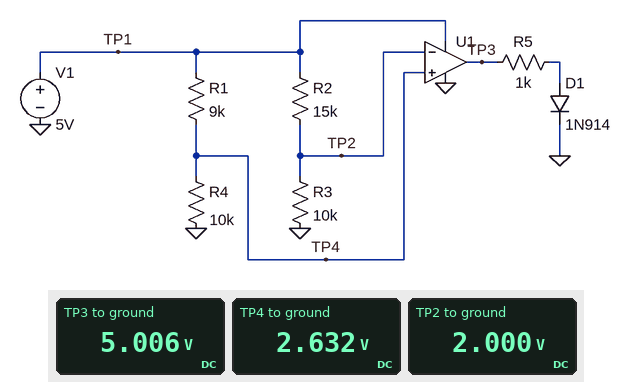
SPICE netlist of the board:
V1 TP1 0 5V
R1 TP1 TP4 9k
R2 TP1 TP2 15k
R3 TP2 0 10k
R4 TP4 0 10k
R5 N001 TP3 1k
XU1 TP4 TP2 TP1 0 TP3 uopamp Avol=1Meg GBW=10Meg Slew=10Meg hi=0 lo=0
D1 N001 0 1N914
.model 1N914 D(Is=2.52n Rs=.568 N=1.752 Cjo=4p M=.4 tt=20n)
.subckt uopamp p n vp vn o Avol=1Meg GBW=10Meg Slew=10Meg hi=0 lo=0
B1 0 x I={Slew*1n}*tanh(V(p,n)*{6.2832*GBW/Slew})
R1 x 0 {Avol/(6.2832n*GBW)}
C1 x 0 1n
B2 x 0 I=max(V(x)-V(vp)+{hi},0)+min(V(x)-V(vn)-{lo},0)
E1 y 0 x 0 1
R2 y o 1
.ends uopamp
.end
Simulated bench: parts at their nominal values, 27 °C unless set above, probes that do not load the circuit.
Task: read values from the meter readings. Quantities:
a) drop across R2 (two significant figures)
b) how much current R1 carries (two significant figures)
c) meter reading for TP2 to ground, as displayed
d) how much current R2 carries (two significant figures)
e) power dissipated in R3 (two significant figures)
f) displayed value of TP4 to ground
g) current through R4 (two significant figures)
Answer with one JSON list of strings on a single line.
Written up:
["3.0 V", "260 µA", "2.000 V", "200 µA", "400 µW", "2.632 V", "260 µA"]
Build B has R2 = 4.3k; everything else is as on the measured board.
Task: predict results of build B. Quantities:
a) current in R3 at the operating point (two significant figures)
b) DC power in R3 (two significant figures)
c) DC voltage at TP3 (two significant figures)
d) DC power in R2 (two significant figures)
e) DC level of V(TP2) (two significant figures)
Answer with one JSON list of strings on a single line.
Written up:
["350 µA", "1.2 mW", "-10 mV", "530 µW", "3.5 V"]
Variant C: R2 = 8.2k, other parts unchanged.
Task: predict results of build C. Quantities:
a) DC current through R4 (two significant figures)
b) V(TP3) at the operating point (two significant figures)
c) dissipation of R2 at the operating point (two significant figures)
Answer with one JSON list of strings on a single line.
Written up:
["260 µA", "-6.2 mV", "620 µW"]
